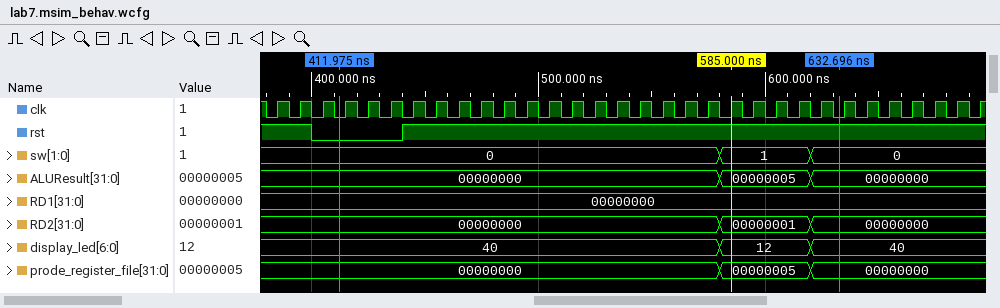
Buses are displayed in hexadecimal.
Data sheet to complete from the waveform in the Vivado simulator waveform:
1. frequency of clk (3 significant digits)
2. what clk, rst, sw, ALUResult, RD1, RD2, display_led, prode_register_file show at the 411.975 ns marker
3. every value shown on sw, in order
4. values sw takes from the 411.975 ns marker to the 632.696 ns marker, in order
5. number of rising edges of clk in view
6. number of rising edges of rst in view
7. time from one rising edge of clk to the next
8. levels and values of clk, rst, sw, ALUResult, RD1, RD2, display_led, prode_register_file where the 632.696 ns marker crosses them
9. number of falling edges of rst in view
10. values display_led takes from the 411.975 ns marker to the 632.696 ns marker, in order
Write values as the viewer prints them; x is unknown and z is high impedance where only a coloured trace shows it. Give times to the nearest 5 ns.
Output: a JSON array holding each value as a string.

["100 MHz", "clk=0, rst=0, sw=0, ALUResult=00000000, RD1=00000000, RD2=00000000, display_led=40, prode_register_file=00000000", "0, 1, 0", "0, 1, 0", "32", "1", "10 ns", "clk=0, rst=1, sw=0, ALUResult=00000000, RD1=00000000, RD2=00000000, display_led=40, prode_register_file=00000000", "1", "40, 12, 40"]
